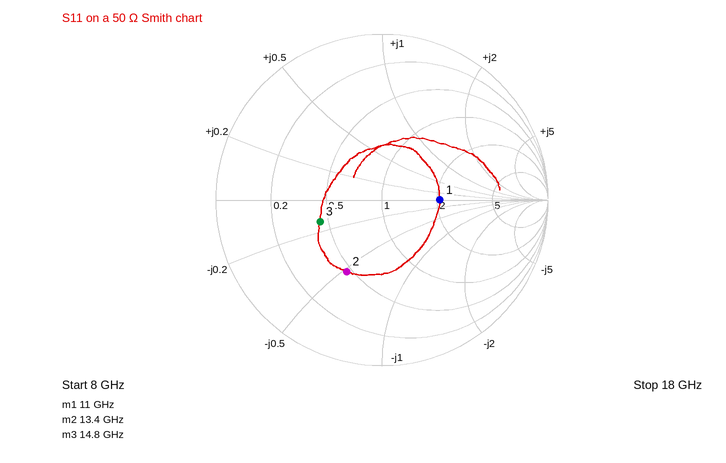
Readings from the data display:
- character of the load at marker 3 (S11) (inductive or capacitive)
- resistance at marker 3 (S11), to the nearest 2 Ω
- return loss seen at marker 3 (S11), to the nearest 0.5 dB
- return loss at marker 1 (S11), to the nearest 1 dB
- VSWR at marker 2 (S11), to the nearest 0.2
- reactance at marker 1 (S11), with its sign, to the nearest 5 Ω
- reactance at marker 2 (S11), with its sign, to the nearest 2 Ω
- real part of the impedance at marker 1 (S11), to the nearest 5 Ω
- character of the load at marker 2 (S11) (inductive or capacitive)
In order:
capacitive
22 Ω
8.0 dB
9 dB
2.8
0 Ω
-26 Ω
105 Ω
capacitive
